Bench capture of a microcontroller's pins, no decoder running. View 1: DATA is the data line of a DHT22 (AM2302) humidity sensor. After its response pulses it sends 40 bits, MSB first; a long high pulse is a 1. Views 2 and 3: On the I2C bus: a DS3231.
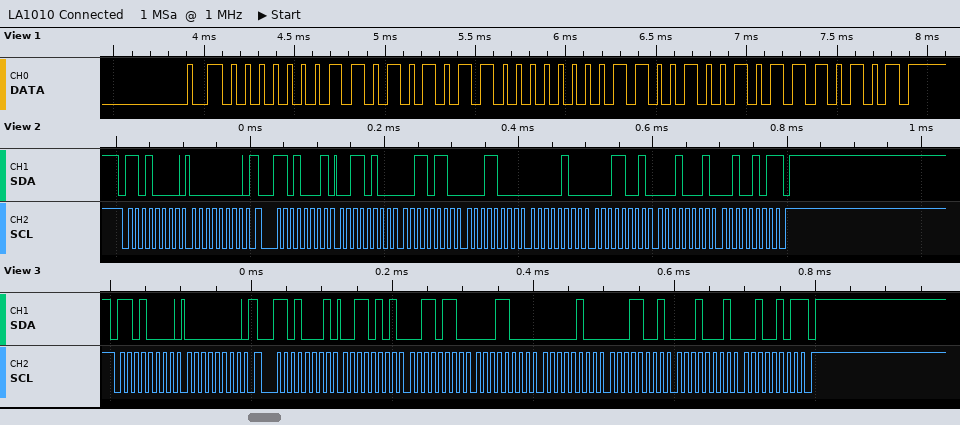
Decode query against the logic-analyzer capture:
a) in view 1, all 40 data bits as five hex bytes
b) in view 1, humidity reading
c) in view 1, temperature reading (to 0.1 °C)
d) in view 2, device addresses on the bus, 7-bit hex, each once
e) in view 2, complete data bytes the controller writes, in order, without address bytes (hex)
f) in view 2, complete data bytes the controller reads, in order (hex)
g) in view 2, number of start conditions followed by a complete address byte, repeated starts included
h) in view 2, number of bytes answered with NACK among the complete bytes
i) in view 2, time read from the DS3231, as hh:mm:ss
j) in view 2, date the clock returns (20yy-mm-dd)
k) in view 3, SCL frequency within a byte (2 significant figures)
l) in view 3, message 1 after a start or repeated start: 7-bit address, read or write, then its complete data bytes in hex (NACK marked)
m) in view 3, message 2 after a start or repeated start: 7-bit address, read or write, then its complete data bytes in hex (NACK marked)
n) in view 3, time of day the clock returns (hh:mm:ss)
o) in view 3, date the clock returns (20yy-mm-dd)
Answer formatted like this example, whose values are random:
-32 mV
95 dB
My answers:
01 AB 00 C9 75
42.7 %
20.1 °C
0x68
00
34 36 18 04 19 11 25
2
1
18:36:34
2025-11-19
100 kHz
0x68 write: 00
0x68 read: 35 36 18 04 19 11 25 NACK
18:36:35
2025-11-19
